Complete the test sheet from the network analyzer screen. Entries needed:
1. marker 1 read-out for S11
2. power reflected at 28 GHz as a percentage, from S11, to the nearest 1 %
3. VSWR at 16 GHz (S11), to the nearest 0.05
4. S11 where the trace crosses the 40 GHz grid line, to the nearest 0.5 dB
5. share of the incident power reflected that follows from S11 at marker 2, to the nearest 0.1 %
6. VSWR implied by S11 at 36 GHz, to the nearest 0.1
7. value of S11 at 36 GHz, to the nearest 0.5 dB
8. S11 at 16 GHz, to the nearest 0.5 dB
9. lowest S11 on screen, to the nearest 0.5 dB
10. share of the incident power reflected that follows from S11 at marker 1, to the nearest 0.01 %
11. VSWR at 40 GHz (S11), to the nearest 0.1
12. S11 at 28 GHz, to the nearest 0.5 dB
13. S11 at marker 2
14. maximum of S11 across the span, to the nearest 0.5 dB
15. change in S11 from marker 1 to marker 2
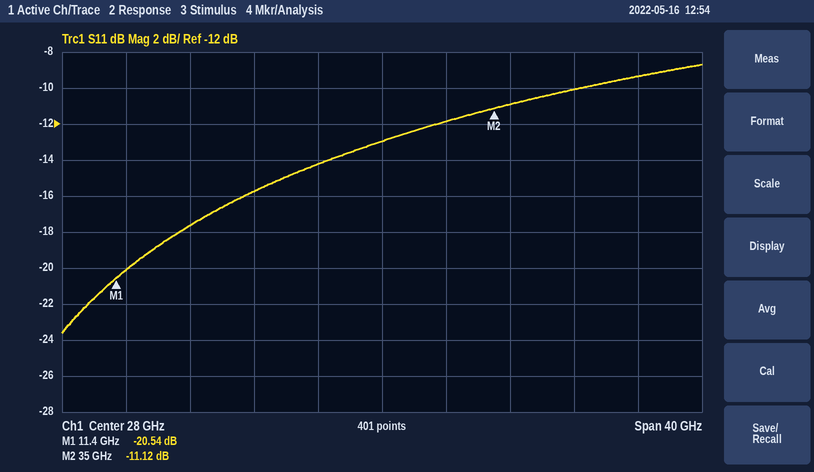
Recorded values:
-20.54 dB
5 %
1.30
-10.0 dB
7.7 %
1.8
-11.0 dB
-17.5 dB
-23.5 dB
0.88 %
1.9
-13.0 dB
-11.12 dB
-8.5 dB
9.42 dB
